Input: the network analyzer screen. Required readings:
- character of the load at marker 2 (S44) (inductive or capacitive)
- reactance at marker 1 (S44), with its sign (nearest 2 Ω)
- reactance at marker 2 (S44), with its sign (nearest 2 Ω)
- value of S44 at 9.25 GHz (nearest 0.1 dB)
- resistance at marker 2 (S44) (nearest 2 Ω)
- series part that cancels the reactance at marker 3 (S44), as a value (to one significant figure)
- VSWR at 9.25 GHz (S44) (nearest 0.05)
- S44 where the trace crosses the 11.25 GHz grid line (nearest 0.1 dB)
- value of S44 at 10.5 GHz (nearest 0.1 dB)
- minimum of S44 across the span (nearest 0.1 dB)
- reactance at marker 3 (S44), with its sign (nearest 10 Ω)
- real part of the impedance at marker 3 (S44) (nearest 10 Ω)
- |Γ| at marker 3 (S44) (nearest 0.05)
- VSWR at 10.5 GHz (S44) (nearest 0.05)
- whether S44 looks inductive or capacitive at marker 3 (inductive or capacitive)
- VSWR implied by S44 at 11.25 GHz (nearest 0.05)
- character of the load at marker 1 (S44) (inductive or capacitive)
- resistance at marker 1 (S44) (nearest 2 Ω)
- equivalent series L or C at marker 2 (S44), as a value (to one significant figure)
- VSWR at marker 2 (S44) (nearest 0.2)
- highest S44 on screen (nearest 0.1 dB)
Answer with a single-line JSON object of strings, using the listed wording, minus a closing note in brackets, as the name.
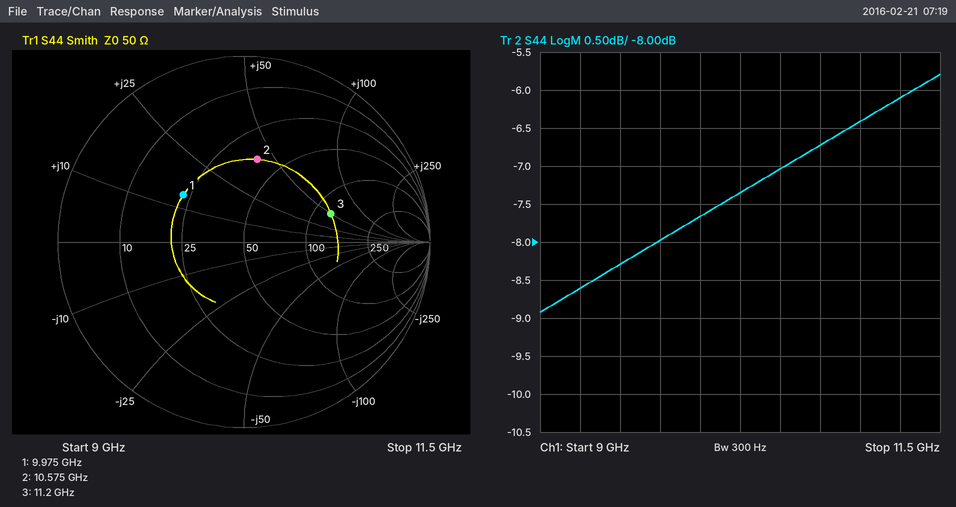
{"character of the load at marker 2 (S44)": "inductive", "reactance at marker 1 (S44), with its sign": "+14 Ω", "reactance at marker 2 (S44), with its sign": "+42 Ω", "value of S44 at 9.25 GHz": "-8.6 dB", "resistance at marker 2 (S44)": "38 Ω", "series part that cancels the reactance at marker 3 (S44), as a value": "300 fF", "VSWR at 9.25 GHz (S44)": "2.20", "S44 where the trace crosses the 11.25 GHz grid line": "-6.1 dB", "value of S44 at 10.5 GHz": "-7.0 dB", "minimum of S44 across the span": "-8.9 dB", "reactance at marker 3 (S44), with its sign": "+50 Ω", "real part of the impedance at marker 3 (S44)": "120 Ω", "|Γ| at marker 3 (S44)": "0.50", "VSWR at 10.5 GHz (S44)": "2.60", "whether S44 looks inductive or capacitive at marker 3": "inductive", "VSWR implied by S44 at 11.25 GHz": "2.95", "character of the load at marker 1 (S44)": "inductive", "resistance at marker 1 (S44)": "22 Ω", "equivalent series L or C at marker 2 (S44), as a value": "600 pH", "VSWR at marker 2 (S44)": "2.6", "highest S44 on screen": "-5.8 dB"}
